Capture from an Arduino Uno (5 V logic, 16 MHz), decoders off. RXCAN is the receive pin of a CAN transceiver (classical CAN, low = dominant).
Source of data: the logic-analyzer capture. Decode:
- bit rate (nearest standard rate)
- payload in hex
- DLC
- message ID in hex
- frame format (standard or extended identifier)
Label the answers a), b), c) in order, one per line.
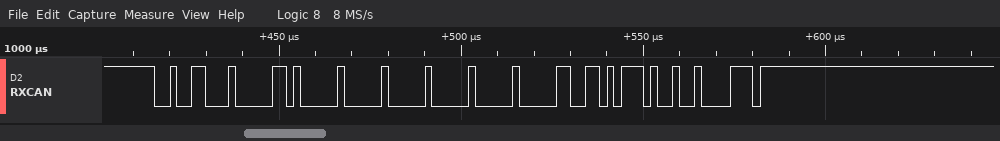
a) 500 kbit/s
b) 00 00 00 02 6B
c) 5
d) 0x262
e) standard
